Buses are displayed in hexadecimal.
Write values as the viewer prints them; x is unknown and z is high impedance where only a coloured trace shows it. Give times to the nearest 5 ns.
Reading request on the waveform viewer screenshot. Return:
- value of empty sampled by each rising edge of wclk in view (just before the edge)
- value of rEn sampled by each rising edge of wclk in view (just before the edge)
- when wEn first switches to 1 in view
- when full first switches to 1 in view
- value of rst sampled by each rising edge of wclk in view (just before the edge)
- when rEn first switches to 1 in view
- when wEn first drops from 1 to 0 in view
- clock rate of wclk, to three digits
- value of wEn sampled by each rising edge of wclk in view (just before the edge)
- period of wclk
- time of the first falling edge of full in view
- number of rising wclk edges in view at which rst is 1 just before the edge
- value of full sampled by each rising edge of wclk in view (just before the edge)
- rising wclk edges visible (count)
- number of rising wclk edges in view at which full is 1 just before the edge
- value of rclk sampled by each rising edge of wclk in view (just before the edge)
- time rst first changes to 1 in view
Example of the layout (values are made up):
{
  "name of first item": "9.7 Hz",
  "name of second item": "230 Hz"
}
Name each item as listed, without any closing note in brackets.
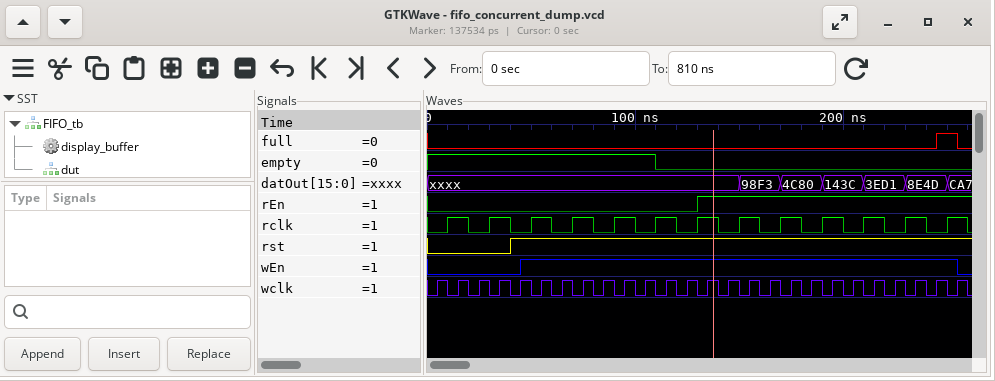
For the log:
{
  "value of empty sampled by each rising edge of wclk in view": "1 1 1 1 1 1 1 1 1 1 1 0 0 0 0 0 0 0 0 0 0 0 0 0 0 0",
  "value of rEn sampled by each rising edge of wclk in view": "0 0 0 0 0 0 0 0 0 0 0 0 0 1 1 1 1 1 1 1 1 1 1 1 1 1",
  "when wEn first switches to 1 in view": "45 ns",
  "when full first switches to 1 in view": "245 ns",
  "value of rst sampled by each rising edge of wclk in view": "0 0 0 0 1 1 1 1 1 1 1 1 1 1 1 1 1 1 1 1 1 1 1 1 1 1",
  "when rEn first switches to 1 in view": "130 ns",
  "when wEn first drops from 1 to 0 in view": "255 ns",
  "clock rate of wclk, to three digits": "100 MHz",
  "value of wEn sampled by each rising edge of wclk in view": "0 0 0 0 0 1 1 1 1 1 1 1 1 1 1 1 1 1 1 1 1 1 1 1 1 1",
  "period of wclk": "10 ns",
  "time of the first falling edge of full in view": "255 ns",
  "number of rising wclk edges in view at which rst is 1 just before the edge": "22",
  "value of full sampled by each rising edge of wclk in view": "0 0 0 0 0 0 0 0 0 0 0 0 0 0 0 0 0 0 0 0 0 0 0 0 0 1",
  "rising wclk edges visible": "26",
  "number of rising wclk edges in view at which full is 1 just before the edge": "1",
  "value of rclk sampled by each rising edge of wclk in view": "0 1 0 1 0 1 0 1 0 1 0 1 0 1 0 1 0 1 0 1 0 1 0 1 0 1",
  "time rst first changes to 1 in view": "40 ns"
}
